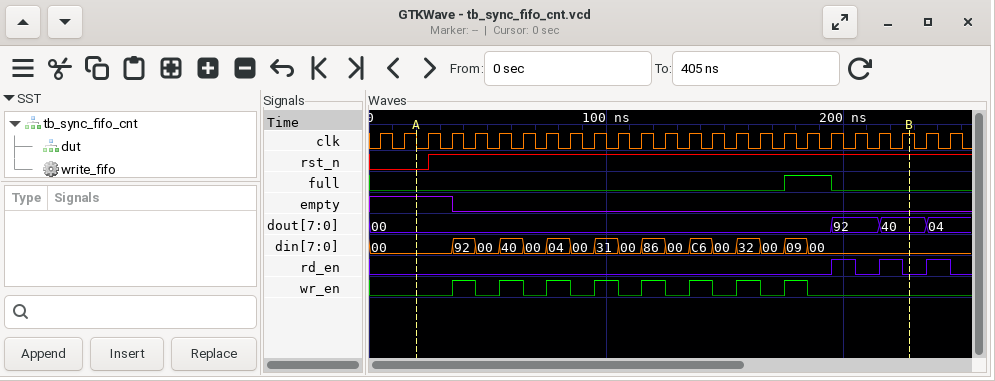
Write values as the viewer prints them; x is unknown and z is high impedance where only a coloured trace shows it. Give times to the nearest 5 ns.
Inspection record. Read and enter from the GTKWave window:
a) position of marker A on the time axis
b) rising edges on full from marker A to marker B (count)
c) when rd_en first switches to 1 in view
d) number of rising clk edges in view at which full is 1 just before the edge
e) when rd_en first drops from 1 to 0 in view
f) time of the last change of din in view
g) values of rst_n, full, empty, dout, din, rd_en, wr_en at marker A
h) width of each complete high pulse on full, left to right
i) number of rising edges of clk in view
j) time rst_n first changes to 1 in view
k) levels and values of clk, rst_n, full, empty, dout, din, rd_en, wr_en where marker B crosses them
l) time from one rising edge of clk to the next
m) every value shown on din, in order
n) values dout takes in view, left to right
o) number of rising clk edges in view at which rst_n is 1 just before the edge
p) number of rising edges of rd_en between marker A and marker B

20 ns
1
195 ns
2
205 ns
185 ns
rst_n=0, full=0, empty=1, dout=00, din=00, rd_en=0, wr_en=0
20 ns
25
25 ns
clk=1, rst_n=1, full=0, empty=0, dout=40, din=00, rd_en=0, wr_en=0
10 ns
00, 92, 00, 40, 00, 04, 00, 31, 00, 86, 00, C6, 00, 32, 00, 09, 00
00, 92, 40, 04
22
2
